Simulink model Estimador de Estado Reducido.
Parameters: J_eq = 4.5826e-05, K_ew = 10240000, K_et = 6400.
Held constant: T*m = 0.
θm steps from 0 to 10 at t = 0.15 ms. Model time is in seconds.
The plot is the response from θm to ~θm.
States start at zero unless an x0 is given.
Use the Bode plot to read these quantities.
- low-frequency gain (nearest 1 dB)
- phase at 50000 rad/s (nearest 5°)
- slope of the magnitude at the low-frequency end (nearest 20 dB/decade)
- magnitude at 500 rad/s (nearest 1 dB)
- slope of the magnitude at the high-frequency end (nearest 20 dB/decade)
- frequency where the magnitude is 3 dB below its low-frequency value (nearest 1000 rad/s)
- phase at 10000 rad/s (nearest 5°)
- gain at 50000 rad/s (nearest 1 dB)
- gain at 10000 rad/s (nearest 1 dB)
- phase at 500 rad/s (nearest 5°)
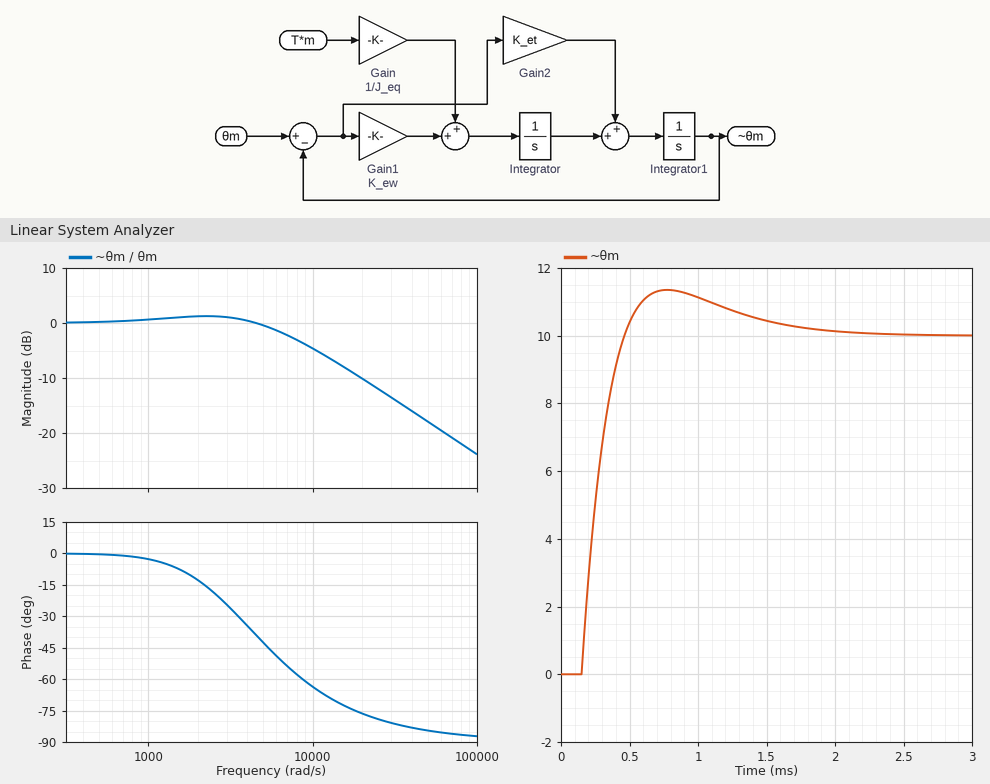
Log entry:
0 dB
-85°
0 dB/decade
0 dB
-20 dB/decade
8000 rad/s
-65°
-18 dB
-5 dB
0°
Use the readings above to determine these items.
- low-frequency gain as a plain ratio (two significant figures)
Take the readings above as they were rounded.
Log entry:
1.0
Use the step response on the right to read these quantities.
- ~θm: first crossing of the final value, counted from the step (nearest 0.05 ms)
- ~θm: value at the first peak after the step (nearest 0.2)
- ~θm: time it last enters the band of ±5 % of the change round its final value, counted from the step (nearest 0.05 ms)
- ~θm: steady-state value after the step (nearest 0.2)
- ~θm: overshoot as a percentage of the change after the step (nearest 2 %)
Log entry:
0.30 ms
11.4
1.30 ms
10.0
14 %
